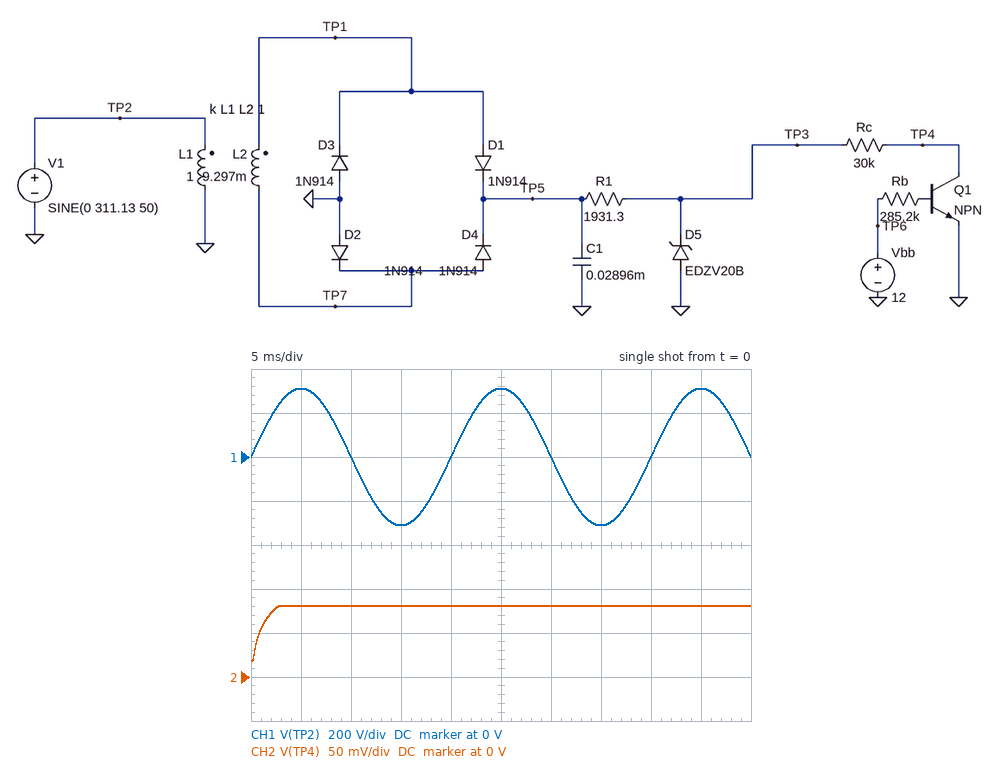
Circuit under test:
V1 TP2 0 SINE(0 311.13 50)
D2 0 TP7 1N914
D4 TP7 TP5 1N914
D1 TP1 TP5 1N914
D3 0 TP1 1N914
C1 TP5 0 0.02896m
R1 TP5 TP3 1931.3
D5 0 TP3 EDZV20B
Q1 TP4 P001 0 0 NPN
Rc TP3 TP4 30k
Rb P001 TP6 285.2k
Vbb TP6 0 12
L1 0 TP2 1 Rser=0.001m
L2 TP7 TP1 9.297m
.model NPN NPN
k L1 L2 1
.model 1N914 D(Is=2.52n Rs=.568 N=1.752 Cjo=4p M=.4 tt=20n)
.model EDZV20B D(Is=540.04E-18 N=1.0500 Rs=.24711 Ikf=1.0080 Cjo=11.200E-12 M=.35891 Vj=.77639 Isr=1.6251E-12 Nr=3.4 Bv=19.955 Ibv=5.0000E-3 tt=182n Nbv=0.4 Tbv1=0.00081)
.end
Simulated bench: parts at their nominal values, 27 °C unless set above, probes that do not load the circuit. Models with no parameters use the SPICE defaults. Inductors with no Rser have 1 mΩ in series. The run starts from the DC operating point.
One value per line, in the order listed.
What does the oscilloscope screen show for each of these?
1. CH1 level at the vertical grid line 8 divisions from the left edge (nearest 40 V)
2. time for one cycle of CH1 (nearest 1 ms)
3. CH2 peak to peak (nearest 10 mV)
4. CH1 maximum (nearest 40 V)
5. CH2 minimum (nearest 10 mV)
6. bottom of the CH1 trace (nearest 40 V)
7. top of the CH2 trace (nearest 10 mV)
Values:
0 V
20 ms
60 mV
320 V
20 mV
-320 V
80 mV
